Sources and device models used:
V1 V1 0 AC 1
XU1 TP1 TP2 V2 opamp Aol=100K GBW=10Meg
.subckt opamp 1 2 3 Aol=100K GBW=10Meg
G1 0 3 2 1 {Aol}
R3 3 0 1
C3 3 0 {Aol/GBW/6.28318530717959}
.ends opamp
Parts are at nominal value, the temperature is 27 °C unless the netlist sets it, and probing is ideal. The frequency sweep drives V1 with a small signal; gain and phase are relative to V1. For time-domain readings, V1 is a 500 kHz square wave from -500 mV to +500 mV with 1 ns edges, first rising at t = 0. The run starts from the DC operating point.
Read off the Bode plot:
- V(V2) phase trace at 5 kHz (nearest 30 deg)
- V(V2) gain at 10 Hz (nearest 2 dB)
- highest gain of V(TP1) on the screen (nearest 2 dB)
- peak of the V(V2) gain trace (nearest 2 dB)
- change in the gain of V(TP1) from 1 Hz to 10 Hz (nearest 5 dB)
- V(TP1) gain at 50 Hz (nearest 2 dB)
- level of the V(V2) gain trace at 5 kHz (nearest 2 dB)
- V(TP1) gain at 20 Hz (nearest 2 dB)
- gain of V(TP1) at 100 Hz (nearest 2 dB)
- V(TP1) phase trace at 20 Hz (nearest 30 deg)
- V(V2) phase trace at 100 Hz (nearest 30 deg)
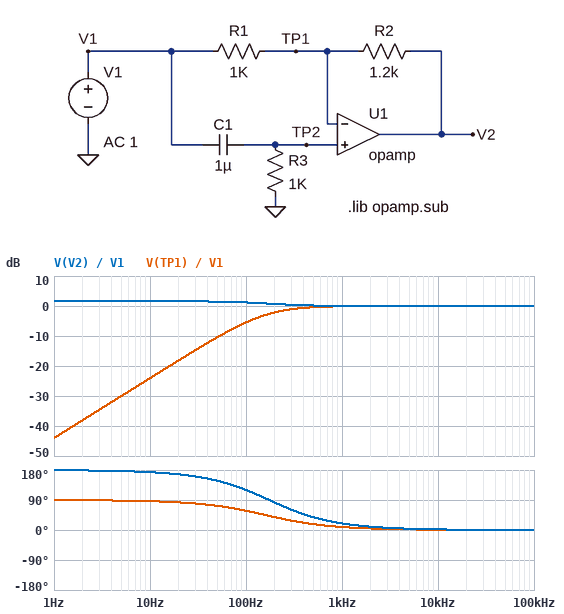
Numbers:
0 deg
2 dB
0 dB
2 dB
20 dB
-10 dB
0 dB
-18 dB
-6 dB
90 deg
120 deg
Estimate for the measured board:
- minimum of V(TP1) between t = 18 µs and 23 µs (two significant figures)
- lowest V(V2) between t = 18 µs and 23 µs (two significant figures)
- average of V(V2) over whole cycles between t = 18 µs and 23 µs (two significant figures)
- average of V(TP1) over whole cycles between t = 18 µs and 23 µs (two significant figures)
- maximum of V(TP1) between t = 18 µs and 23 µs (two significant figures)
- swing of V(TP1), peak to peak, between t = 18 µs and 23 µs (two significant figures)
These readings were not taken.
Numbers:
-11 mV
580 mV
1.1 V
490 mV
990 mV
1.0 V
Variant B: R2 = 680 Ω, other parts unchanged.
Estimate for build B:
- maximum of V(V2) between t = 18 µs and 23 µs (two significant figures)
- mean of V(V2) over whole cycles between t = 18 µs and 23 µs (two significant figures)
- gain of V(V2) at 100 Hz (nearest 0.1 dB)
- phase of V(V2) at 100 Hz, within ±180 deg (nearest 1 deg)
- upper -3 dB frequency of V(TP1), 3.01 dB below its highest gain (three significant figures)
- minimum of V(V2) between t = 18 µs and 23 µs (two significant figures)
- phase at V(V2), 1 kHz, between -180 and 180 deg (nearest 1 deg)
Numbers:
1.3 V
820 mV
-2.1 dB
105 deg
7.26 MHz
320 mV
15 deg
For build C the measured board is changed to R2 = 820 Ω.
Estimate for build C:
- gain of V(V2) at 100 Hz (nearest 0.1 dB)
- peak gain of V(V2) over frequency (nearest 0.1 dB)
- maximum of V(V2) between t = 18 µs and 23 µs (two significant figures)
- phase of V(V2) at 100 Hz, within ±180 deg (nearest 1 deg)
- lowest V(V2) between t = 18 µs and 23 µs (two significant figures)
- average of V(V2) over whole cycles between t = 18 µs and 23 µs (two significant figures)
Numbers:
-1.2 dB
0 dB
1.4 V
110 deg
390 mV
890 mV
